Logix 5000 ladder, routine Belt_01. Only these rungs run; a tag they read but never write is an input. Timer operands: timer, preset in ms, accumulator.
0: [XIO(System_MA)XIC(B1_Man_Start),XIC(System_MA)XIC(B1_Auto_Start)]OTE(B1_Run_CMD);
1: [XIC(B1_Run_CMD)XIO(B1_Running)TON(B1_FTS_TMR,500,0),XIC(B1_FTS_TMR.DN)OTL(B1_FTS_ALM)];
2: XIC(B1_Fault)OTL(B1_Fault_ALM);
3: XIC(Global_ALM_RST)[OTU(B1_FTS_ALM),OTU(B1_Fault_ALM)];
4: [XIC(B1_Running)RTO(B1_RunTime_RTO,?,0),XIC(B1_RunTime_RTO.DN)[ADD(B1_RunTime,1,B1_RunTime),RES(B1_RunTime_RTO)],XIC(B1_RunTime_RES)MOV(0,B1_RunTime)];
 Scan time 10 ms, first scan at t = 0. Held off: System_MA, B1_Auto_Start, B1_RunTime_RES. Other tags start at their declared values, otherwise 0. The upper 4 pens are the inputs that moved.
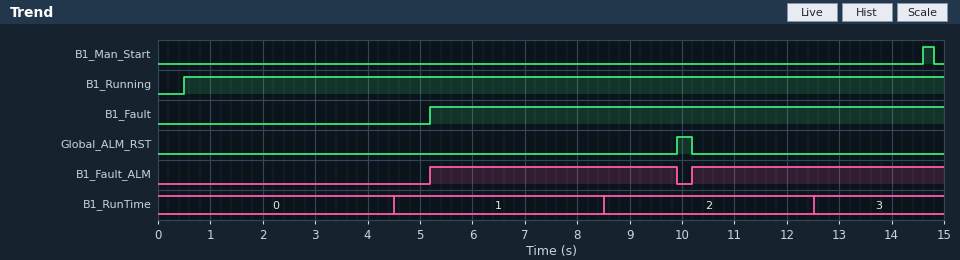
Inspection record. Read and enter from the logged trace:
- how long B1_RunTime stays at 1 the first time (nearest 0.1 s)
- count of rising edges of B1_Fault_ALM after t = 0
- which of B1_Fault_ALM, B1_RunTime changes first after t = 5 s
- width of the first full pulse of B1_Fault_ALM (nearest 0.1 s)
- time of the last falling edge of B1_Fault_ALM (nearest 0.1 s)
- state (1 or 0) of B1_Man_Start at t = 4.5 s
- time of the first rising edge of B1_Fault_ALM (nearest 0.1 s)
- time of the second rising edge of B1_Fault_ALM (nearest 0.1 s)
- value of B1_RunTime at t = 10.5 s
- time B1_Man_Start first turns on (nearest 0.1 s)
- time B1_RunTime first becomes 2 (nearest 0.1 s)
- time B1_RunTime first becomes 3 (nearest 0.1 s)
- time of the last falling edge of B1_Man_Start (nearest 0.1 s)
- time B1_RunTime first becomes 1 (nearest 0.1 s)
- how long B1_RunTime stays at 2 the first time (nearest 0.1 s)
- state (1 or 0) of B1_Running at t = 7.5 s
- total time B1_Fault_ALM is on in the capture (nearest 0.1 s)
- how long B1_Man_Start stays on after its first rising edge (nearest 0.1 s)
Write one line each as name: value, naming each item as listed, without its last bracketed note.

how long B1_RunTime stays at 1 the first time: 4.0 s
count of rising edges of B1_Fault_ALM after t = 0: 2
which of B1_Fault_ALM, B1_RunTime changes first after t = 5 s: B1_Fault_ALM
width of the first full pulse of B1_Fault_ALM: 4.7 s
time of the last falling edge of B1_Fault_ALM: 9.9 s
state (1 or 0) of B1_Man_Start at t = 4.5 s: 0
time of the first rising edge of B1_Fault_ALM: 5.2 s
time of the second rising edge of B1_Fault_ALM: 10.2 s
value of B1_RunTime at t = 10.5 s: 2
time B1_Man_Start first turns on: 14.6 s
time B1_RunTime first becomes 2: 8.5 s
time B1_RunTime first becomes 3: 12.5 s
time of the last falling edge of B1_Man_Start: 14.8 s
time B1_RunTime first becomes 1: 4.5 s
how long B1_RunTime stays at 2 the first time: 4.0 s
state (1 or 0) of B1_Running at t = 7.5 s: 1
total time B1_Fault_ALM is on in the capture: 9.5 s
how long B1_Man_Start stays on after its first rising edge: 0.2 s
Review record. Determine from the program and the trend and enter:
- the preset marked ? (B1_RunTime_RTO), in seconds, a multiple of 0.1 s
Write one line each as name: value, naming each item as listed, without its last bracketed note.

the preset marked ? (B1_RunTime_RTO), in seconds, a multiple of 0.1 s: 4.0 s
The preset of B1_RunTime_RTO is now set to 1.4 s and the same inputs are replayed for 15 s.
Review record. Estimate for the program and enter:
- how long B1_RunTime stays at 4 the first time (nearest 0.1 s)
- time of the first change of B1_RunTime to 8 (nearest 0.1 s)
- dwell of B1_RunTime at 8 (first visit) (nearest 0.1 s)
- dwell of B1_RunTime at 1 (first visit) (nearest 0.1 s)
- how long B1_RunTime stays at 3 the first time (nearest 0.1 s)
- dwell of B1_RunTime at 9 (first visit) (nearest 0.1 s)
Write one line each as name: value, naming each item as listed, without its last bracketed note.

how long B1_RunTime stays at 4 the first time: 1.4 s
time of the first change of B1_RunTime to 8: 11.8 s
dwell of B1_RunTime at 8 (first visit): 1.4 s
dwell of B1_RunTime at 1 (first visit): 1.4 s
how long B1_RunTime stays at 3 the first time: 1.4 s
dwell of B1_RunTime at 9 (first visit): 1.4 s
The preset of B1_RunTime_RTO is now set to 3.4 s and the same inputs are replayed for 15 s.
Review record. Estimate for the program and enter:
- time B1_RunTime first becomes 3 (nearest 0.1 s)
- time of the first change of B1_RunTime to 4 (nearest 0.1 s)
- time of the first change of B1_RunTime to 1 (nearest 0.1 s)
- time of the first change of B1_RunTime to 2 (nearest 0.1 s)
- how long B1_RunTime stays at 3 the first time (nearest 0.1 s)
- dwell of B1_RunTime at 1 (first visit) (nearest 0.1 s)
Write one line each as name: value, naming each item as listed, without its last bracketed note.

time B1_RunTime first becomes 3: 10.7 s
time of the first change of B1_RunTime to 4: 14.1 s
time of the first change of B1_RunTime to 1: 3.9 s
time of the first change of B1_RunTime to 2: 7.3 s
how long B1_RunTime stays at 3 the first time: 3.4 s
dwell of B1_RunTime at 1 (first visit): 3.4 s
